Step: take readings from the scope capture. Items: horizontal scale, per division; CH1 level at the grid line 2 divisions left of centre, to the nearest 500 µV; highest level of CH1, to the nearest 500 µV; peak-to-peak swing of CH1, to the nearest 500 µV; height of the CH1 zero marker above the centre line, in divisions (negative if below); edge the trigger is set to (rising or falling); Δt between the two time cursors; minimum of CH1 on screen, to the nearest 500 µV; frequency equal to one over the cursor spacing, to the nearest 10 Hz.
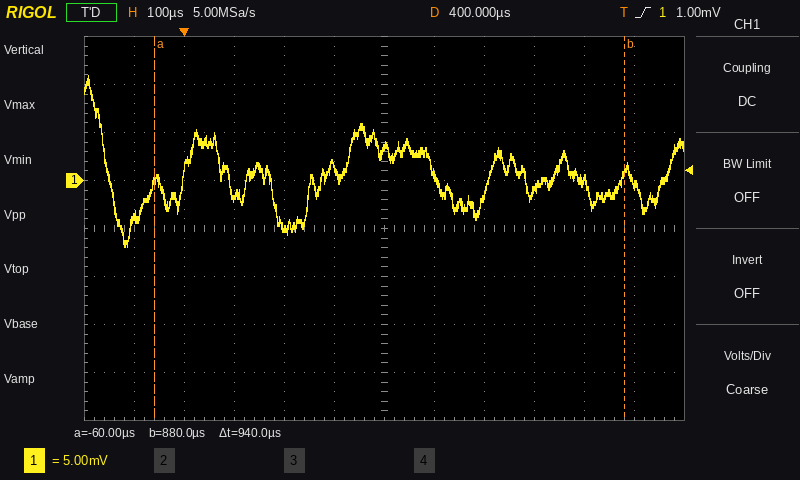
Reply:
100 µs
-5.0 mV
11.0 mV
18.0 mV
+1.0 div
rising
940 µs
-7.0 mV
1.06 kHz
